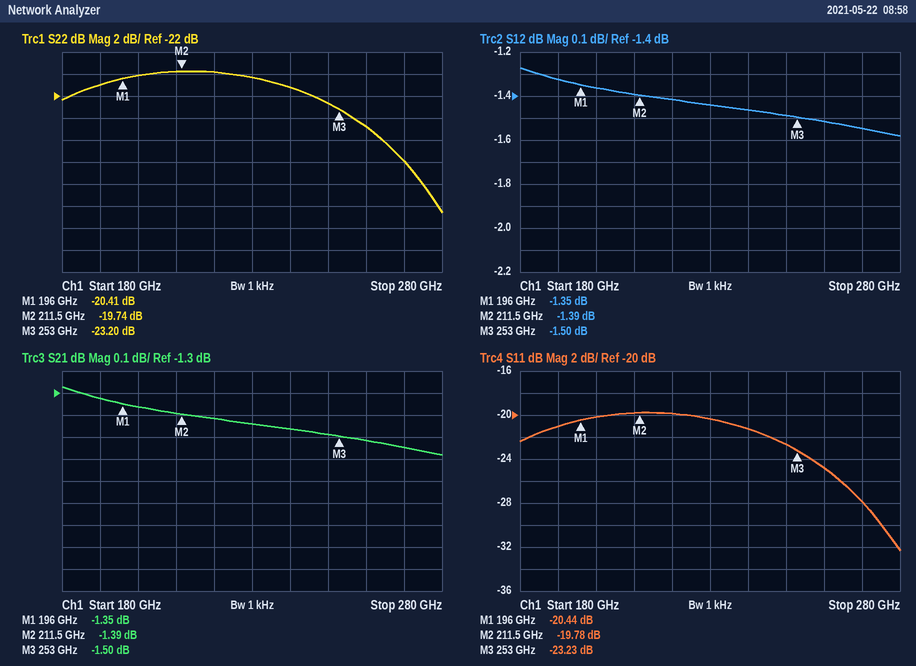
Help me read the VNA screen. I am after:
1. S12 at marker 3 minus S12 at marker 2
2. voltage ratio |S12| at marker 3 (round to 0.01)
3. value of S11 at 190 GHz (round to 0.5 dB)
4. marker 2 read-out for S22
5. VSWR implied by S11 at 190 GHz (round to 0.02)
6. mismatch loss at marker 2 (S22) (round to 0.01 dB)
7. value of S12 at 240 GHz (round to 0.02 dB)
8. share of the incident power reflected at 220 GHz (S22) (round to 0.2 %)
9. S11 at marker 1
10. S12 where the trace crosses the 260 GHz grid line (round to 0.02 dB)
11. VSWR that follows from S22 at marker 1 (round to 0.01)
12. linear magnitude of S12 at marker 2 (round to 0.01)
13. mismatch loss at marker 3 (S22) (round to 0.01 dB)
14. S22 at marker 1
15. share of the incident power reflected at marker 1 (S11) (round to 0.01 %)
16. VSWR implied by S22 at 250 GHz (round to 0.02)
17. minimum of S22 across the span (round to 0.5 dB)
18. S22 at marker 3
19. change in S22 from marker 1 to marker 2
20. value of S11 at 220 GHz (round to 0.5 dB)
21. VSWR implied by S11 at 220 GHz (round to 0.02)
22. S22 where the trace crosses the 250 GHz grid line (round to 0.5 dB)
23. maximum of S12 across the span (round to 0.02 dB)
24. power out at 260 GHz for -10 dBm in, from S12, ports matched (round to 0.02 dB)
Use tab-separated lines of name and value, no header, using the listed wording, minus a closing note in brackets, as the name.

S12 at marker 3 minus S12 at marker 2	-0.11 dB
voltage ratio |S12| at marker 3	0.84
value of S11 at 190 GHz	-21.0 dB
marker 2 read-out for S22	-19.74 dB
VSWR implied by S11 at 190 GHz	1.20
mismatch loss at marker 2 (S22)	0.05 dB
value of S12 at 240 GHz	-1.46 dB
share of the incident power reflected at 220 GHz (S22)	1.0 %
S11 at marker 1	-20.44 dB
S12 where the trace crosses the 260 GHz grid line	-1.52 dB
VSWR that follows from S22 at marker 1	1.21
linear magnitude of S12 at marker 2	0.85
mismatch loss at marker 3 (S22)	0.02 dB
S22 at marker 1	-20.41 dB
share of the incident power reflected at marker 1 (S11)	0.90 %
VSWR implied by S22 at 250 GHz	1.16
minimum of S22 across the span	-32.5 dB
S22 at marker 3	-23.20 dB
change in S22 from marker 1 to marker 2	0.67 dB
value of S11 at 220 GHz	-20.0 dB
VSWR implied by S11 at 220 GHz	1.22
S22 where the trace crosses the 250 GHz grid line	-22.5 dB
maximum of S12 across the span	-1.28 dB
power out at 260 GHz for -10 dBm in, from S12, ports matched	-11.52 dBm
